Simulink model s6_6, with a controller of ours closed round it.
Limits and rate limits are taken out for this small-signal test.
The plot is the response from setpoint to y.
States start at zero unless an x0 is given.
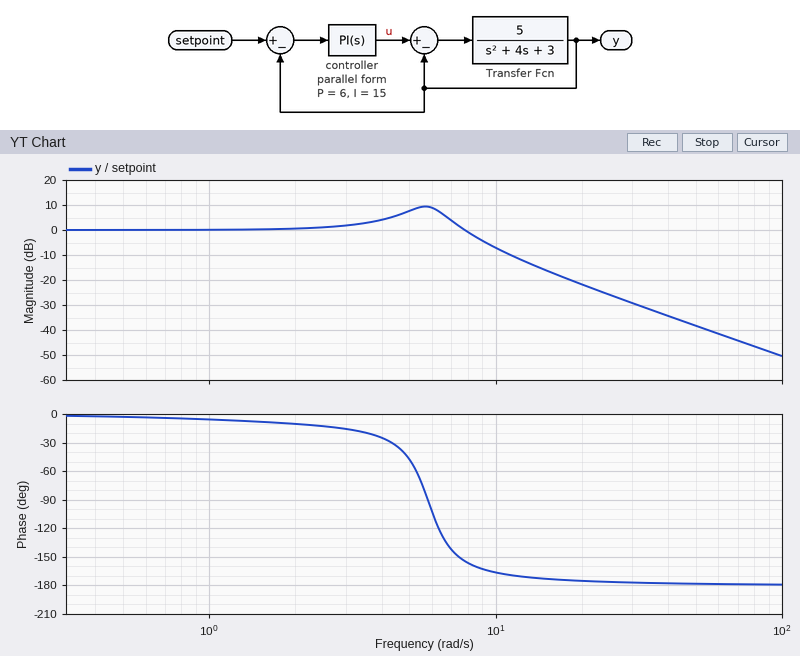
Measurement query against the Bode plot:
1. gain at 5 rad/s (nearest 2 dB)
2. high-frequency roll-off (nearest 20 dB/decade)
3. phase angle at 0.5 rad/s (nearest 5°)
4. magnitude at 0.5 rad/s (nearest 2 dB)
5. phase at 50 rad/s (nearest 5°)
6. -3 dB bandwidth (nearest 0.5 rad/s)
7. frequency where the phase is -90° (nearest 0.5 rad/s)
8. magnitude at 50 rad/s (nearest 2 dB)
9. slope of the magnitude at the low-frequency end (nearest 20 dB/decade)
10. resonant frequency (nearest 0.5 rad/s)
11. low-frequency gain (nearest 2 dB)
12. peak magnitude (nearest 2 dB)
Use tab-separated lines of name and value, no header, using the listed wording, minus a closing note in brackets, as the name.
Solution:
gain at 5 rad/s	8 dB
high-frequency roll-off	-40 dB/decade
phase angle at 0.5 rad/s	-5°
magnitude at 0.5 rad/s	0 dB
phase at 50 rad/s	-180°
-3 dB bandwidth	8.5 rad/s
frequency where the phase is -90°	6.0 rad/s
magnitude at 50 rad/s	-38 dB
slope of the magnitude at the low-frequency end	0 dB/decade
resonant frequency	5.5 rad/s
low-frequency gain	0 dB
peak magnitude	10 dB
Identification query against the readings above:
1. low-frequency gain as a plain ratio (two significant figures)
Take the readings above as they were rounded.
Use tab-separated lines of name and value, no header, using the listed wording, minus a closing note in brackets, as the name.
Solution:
low-frequency gain as a plain ratio	1.0
